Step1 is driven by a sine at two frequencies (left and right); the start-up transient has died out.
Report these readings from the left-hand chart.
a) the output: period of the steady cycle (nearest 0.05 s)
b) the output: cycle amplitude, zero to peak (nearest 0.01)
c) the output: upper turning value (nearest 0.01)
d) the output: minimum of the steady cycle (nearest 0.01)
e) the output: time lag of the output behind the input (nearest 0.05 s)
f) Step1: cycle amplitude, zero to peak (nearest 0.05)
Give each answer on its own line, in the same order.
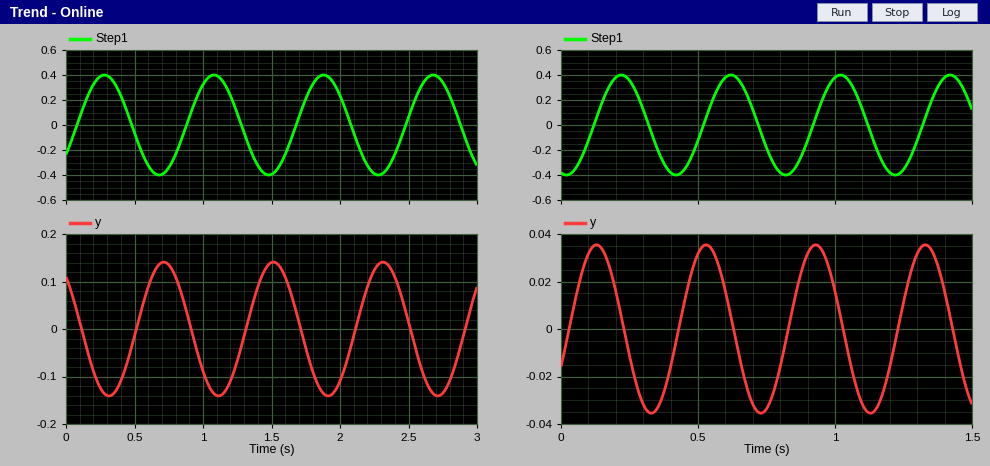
0.80 s
0.14
0.14
-0.14
0.45 s
0.40
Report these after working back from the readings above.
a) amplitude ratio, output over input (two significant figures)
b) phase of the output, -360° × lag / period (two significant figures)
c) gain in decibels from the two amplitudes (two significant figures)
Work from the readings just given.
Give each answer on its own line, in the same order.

0.35
-200°
-9.1 dB
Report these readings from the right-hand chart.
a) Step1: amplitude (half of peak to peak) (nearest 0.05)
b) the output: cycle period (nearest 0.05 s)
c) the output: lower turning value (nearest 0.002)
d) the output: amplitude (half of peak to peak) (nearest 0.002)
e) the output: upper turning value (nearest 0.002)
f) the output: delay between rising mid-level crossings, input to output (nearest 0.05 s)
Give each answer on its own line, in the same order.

0.40
0.40 s
-0.036
0.036
0.036
0.30 s
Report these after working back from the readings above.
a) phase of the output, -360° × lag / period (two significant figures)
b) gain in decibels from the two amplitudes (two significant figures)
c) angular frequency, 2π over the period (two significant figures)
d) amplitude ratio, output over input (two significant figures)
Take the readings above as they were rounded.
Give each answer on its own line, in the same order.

-270°
-21 dB
16 rad/s
0.090
